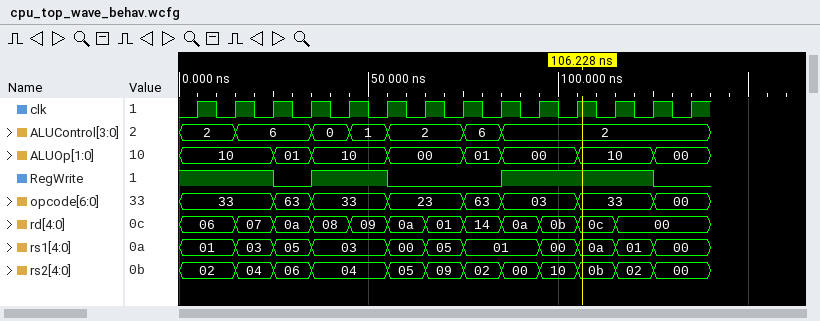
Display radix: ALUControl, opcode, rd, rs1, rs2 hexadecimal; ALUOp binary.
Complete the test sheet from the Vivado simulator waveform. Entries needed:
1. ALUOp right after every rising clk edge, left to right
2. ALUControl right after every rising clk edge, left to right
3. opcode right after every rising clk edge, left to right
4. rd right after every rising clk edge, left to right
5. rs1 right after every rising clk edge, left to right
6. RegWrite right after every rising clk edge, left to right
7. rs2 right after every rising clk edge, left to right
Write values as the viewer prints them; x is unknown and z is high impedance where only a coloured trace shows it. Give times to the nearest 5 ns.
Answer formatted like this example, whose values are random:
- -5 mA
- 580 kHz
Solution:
- 10, 10, 01, 10, 10, 00, 00, 01, 00, 00, 10, 10, 00, 00
- 2, 6, 6, 0, 1, 2, 2, 6, 2, 2, 2, 2, 2, 2
- 33, 33, 63, 33, 33, 23, 23, 63, 03, 03, 33, 33, 00, 00
- 06, 07, 0a, 08, 09, 0a, 01, 14, 0a, 0b, 0c, 00, 00, 00
- 01, 03, 05, 03, 03, 00, 05, 01, 01, 00, 0a, 01, 00, 00
- 1 1 0 1 1 0 0 0 1 1 1 1 0 0
- 02, 04, 06, 04, 04, 05, 09, 02, 00, 10, 0b, 02, 00, 00
